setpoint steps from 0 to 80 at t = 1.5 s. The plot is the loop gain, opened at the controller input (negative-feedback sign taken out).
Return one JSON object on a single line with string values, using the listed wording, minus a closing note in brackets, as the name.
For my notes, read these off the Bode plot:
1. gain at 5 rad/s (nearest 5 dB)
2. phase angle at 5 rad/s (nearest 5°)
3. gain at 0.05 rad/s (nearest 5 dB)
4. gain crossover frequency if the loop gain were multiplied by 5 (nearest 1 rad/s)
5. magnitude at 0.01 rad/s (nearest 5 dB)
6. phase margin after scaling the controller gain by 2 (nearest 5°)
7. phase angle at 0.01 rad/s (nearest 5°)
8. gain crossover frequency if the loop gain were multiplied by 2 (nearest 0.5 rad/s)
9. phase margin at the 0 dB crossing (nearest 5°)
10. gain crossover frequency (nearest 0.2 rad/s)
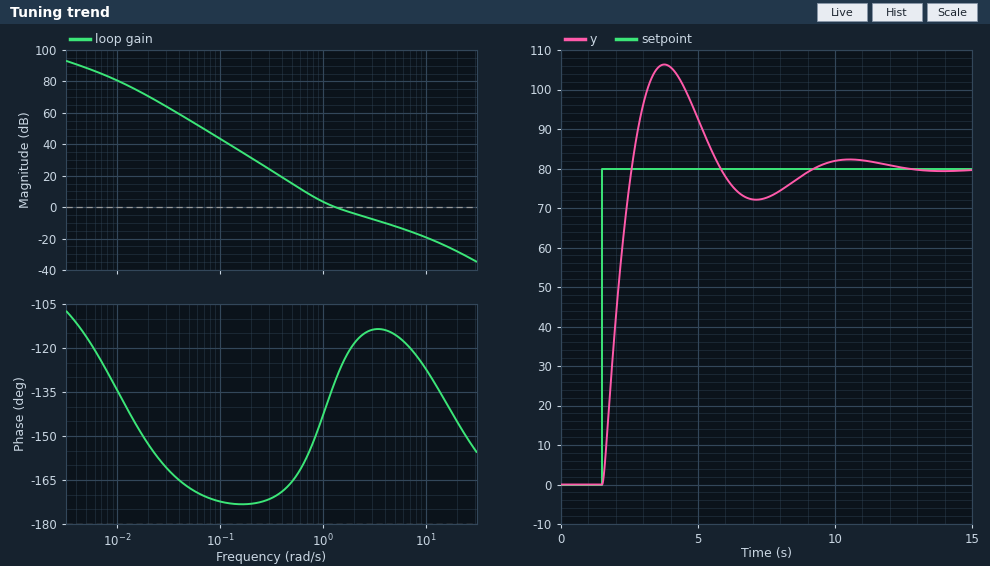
{"gain at 5 rad/s": "-10 dB", "phase angle at 5 rad/s": "-115°", "gain at 0.05 rad/s": "55 dB", "gain crossover frequency if the loop gain were multiplied by 5": "6 rad/s", "magnitude at 0.01 rad/s": "80 dB", "phase margin after scaling the controller gain by 2": "65°", "phase angle at 0.01 rad/s": "-135°", "gain crossover frequency if the loop gain were multiplied by 2": "2.5 rad/s", "phase margin at the 0 dB crossing": "50°", "gain crossover frequency": "1.4 rad/s"}
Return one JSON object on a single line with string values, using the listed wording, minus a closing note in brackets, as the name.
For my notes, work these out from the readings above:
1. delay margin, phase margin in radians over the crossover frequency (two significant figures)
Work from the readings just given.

{"delay margin, phase margin in radians over the crossover frequency": "0.62 s"}
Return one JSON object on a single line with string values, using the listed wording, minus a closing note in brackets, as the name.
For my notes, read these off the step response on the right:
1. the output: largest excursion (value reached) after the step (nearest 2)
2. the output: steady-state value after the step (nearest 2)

{"the output: largest excursion (value reached) after the step": "106", "the output: steady-state value after the step": "80"}
